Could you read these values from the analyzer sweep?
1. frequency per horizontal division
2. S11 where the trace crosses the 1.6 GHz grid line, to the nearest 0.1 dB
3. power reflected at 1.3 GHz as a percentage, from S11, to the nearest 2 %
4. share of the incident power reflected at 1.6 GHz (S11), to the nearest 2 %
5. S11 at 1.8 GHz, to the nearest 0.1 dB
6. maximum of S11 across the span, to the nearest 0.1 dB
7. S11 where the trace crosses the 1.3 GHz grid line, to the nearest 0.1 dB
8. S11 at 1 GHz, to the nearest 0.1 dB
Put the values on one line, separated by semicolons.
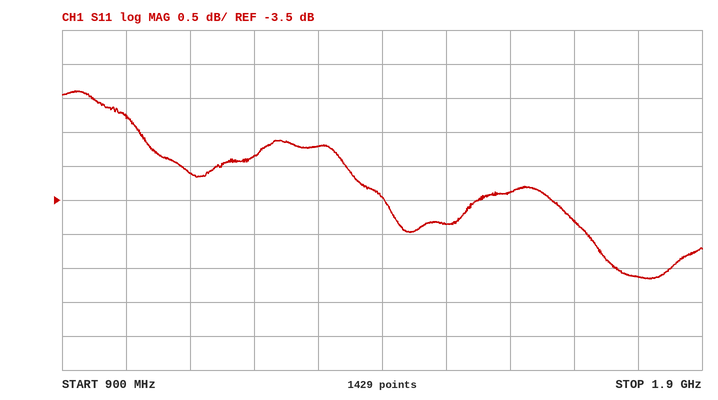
100 MHz; -3.4 dB; 54 %; 46 %; -4.6 dB; -1.9 dB; -2.7 dB; -2.3 dB
